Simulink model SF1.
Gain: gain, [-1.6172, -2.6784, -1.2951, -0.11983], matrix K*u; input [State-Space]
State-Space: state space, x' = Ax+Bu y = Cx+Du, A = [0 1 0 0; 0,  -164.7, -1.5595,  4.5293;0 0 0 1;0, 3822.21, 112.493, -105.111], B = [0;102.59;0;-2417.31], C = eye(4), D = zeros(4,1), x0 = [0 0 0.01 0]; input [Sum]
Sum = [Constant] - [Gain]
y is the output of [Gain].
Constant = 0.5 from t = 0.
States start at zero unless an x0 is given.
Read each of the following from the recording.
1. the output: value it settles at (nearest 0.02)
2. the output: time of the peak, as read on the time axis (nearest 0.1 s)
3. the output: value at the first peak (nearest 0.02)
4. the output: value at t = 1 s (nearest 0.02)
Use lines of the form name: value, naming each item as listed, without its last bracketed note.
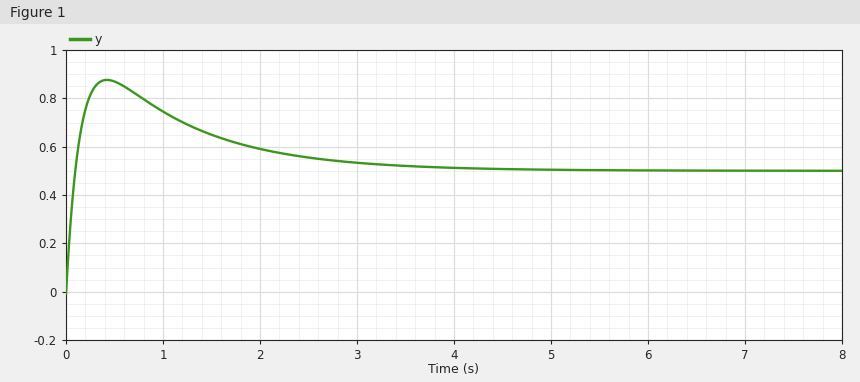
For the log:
the output: value it settles at: 0.50
the output: time of the peak, as read on the time axis: 0.4 s
the output: value at the first peak: 0.88
the output: value at t = 1 s: 0.74
